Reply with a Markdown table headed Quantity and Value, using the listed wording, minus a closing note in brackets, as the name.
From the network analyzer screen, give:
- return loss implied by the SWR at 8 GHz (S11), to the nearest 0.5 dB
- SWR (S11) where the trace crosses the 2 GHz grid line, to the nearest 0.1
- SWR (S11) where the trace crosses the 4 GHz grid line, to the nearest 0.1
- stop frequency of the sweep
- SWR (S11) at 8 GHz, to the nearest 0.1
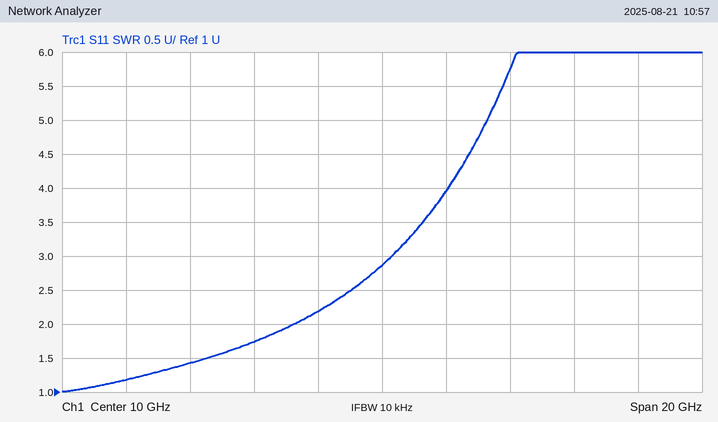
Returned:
| Quantity | Value |
|---|---|
| return loss implied by the SWR at 8 GHz (S11), to the nearest 0.5 dB | 8.5 dB |
| SWR (S11) where the trace crosses the 2 GHz grid line, to the nearest 0.1 | 1.2 |
| SWR (S11) where the trace crosses the 4 GHz grid line, to the nearest 0.1 | 1.4 |
| stop frequency of the sweep | 20 GHz |
| SWR (S11) at 8 GHz, to the nearest 0.1 | 2.2 |
